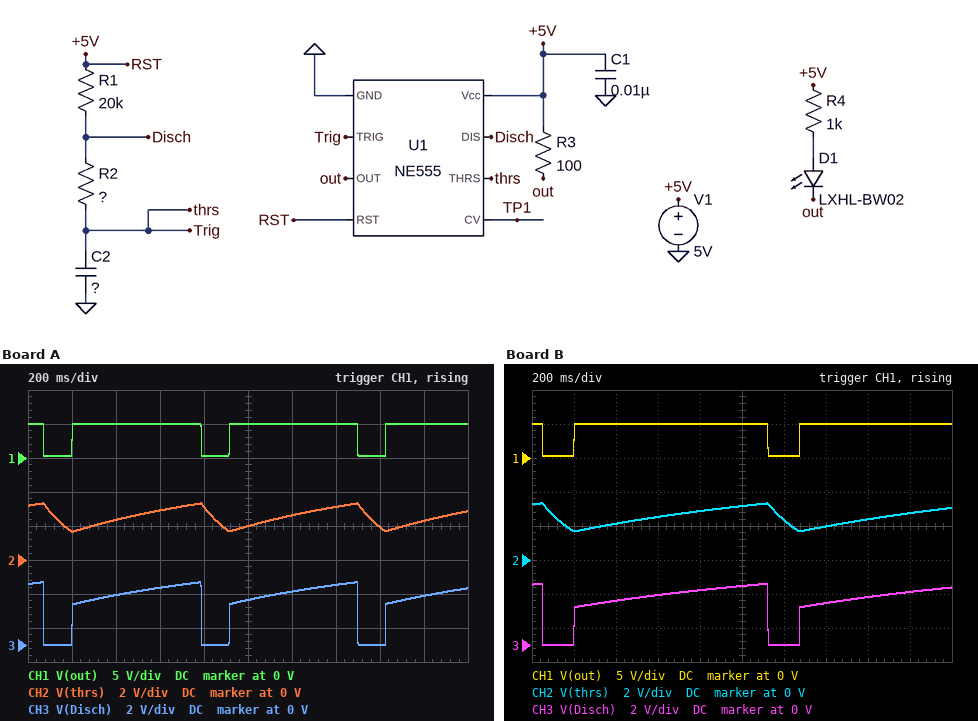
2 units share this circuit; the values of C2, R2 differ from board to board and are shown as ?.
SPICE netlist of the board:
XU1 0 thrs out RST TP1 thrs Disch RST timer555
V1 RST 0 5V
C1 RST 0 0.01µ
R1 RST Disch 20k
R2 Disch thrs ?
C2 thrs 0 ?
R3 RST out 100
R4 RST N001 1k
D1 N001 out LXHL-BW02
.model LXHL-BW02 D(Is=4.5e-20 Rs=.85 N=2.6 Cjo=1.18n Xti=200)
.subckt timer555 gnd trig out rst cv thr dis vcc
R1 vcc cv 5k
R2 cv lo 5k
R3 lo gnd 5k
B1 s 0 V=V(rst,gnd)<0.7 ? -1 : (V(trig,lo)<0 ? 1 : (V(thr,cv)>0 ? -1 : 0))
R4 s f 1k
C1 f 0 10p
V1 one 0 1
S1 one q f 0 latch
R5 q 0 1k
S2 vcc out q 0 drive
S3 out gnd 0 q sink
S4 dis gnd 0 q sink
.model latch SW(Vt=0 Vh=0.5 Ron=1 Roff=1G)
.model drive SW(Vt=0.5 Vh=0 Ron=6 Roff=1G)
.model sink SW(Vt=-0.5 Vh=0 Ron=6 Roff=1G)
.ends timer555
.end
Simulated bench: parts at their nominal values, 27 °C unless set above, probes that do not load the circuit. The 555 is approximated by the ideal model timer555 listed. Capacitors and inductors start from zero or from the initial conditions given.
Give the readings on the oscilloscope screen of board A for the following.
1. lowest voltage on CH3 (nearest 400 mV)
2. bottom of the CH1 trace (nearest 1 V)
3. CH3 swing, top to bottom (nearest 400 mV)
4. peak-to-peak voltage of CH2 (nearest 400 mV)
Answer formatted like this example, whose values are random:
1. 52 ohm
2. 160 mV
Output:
1. 0 V
2. 0 V
3. 3.6 V
4. 1.6 V
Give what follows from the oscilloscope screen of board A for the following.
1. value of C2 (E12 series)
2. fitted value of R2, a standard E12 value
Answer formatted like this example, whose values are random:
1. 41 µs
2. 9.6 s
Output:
1. 33 µF
2. 5.6 kΩ
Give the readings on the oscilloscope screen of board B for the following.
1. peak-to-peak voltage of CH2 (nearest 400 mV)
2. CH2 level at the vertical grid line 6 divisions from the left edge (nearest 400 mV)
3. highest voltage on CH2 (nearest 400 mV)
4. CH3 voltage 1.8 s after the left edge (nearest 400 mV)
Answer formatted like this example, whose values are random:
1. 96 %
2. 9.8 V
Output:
1. 1.6 V
2. 2.4 V
3. 3.2 V
4. 3.2 V
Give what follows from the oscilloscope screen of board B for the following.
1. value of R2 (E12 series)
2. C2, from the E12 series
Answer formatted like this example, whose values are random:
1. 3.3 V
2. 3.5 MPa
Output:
1. 3.9 kΩ
2. 56 µF
